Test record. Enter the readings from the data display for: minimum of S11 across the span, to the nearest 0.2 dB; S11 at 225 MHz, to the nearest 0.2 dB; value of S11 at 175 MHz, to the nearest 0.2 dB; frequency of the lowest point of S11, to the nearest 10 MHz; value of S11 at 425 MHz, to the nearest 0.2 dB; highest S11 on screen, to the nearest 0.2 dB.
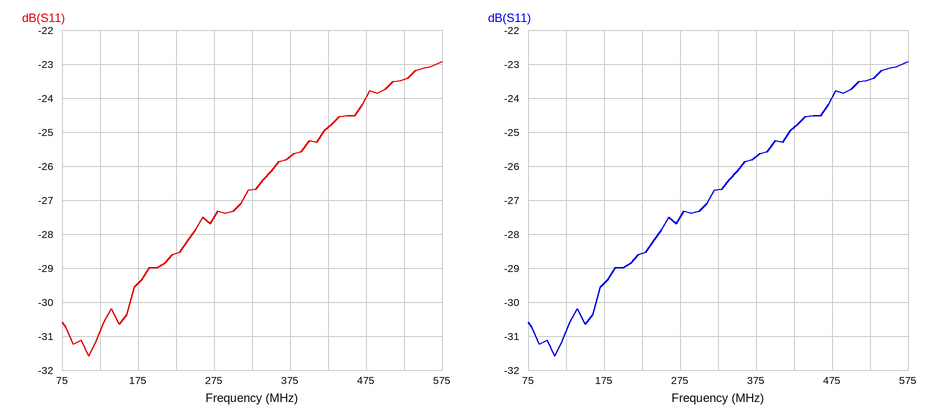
-31.6 dB
-28.6 dB
-29.4 dB
110 MHz
-24.8 dB
-23.0 dB
